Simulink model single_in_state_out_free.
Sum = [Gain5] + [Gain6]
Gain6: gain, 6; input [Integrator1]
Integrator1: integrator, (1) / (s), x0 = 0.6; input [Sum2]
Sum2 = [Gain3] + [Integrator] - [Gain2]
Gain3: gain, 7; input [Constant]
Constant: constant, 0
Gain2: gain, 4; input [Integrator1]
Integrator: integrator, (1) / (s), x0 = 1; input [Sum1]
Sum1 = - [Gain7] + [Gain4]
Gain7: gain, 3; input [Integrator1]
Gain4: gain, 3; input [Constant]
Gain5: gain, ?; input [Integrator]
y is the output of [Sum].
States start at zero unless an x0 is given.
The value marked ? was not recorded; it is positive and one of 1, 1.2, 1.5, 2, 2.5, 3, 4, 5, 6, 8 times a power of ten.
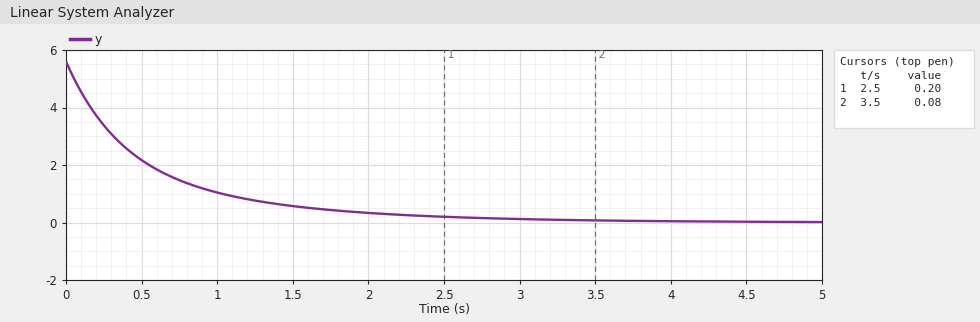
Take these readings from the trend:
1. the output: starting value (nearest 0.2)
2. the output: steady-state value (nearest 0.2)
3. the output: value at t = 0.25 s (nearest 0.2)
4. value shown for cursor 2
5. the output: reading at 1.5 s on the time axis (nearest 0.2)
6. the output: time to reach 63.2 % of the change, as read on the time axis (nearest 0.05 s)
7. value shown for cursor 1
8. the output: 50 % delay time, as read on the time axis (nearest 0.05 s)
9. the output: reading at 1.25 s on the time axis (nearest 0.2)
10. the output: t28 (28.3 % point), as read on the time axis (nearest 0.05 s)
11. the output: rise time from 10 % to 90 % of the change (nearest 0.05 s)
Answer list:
5.6
0.0
3.4
0.08
0.6
0.55 s
0.20
0.35 s
0.8
0.15 s
1.45 s
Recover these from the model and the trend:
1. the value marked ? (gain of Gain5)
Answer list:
2
